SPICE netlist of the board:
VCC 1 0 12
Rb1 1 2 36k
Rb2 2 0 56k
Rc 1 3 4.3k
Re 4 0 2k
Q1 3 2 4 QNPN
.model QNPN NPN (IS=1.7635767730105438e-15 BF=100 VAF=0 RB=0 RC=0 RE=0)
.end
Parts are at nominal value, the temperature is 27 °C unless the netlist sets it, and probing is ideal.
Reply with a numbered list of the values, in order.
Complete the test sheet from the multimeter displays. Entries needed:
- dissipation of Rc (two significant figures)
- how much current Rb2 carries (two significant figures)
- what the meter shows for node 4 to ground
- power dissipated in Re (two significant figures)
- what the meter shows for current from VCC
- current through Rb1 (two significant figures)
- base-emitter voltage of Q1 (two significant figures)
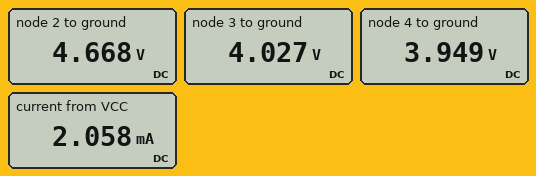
1. 15 mW
2. 83 µA
3. 3.949 V
4. 7.8 mW
5. 2.058 mA
6. 200 µA
7. 720 mV
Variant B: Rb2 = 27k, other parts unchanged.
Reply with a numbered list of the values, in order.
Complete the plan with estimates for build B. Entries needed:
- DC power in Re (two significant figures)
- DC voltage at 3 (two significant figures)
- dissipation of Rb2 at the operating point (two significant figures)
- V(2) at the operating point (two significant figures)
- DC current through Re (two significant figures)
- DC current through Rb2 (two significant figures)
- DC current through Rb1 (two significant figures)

1. 7.3 mW
2. 3.9 V
3. 760 µW
4. 4.5 V
5. 1.9 mA
6. 170 µA
7. 210 µA
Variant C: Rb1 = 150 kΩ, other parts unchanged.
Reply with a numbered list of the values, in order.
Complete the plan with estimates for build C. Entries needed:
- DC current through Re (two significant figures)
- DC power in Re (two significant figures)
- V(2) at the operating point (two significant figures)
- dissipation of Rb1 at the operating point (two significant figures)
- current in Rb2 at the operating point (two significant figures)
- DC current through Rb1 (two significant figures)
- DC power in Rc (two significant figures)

1. 1.1 mA
2. 2.3 mW
3. 2.8 V
4. 560 µW
5. 51 µA
6. 61 µA
7. 4.8 mW
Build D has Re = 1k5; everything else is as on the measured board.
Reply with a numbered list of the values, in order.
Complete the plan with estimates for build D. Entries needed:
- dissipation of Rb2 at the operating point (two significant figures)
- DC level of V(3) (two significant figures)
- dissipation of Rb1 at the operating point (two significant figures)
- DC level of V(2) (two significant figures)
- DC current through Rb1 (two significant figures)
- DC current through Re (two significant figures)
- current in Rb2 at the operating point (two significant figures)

1. 280 µW
2. 3.3 V
3. 1.8 mW
4. 4.0 V
5. 220 µA
6. 2.2 mA
7. 71 µA
